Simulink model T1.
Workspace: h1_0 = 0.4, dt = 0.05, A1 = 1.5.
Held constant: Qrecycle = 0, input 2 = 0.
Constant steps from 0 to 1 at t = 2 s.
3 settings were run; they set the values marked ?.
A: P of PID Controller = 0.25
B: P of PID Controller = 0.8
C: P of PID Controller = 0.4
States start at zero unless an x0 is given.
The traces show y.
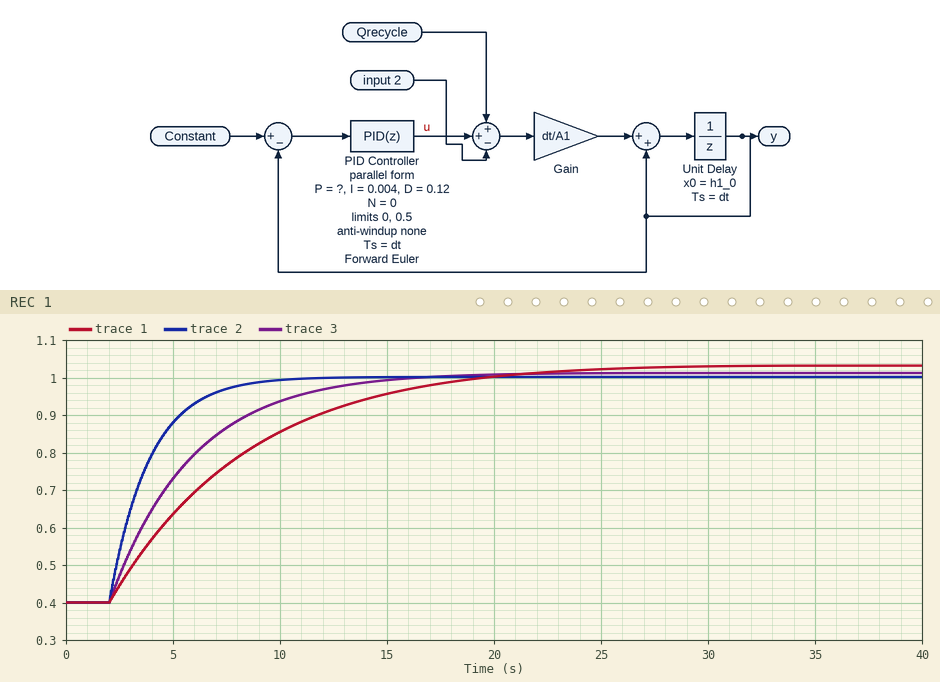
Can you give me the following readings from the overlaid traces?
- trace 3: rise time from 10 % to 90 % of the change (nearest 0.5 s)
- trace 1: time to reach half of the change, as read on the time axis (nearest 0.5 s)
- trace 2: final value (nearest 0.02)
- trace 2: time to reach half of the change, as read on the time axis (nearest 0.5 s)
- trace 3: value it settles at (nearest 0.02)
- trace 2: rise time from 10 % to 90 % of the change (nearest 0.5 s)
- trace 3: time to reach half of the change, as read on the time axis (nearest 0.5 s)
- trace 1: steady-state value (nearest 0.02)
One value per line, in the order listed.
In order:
8.5 s
6.5 s
1.00
3.5 s
1.02
4.0 s
4.5 s
1.04
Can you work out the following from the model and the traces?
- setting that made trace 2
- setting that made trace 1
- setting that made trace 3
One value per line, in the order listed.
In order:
B
A
C
